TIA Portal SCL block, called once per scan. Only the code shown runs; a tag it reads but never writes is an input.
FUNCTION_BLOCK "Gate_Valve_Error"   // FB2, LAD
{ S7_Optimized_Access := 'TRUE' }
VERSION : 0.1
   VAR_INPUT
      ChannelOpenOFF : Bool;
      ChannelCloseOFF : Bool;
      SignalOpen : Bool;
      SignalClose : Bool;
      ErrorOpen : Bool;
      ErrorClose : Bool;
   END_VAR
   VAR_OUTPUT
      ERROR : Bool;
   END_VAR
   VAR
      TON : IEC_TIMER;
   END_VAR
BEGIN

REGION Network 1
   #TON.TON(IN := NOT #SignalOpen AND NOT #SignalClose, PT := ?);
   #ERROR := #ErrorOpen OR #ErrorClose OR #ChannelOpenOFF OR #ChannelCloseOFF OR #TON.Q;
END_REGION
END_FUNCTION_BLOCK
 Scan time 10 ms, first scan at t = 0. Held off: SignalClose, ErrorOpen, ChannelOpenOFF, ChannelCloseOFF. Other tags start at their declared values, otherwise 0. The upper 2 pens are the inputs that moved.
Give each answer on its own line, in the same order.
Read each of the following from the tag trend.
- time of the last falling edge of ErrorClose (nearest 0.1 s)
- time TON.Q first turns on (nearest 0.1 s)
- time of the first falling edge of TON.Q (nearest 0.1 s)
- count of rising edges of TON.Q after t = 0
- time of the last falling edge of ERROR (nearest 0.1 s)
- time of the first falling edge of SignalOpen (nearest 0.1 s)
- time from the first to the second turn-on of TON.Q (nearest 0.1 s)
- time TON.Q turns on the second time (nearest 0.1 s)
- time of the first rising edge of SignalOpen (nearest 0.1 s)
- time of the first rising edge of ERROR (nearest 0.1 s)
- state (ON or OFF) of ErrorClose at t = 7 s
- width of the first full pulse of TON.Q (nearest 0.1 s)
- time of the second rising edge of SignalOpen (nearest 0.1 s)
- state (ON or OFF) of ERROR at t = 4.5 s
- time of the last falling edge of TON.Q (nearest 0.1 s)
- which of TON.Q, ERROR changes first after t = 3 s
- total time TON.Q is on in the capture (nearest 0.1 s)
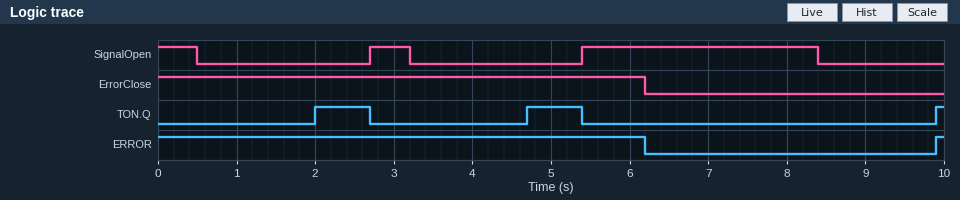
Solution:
6.2 s
2.0 s
2.7 s
3
6.2 s
0.5 s
2.7 s
4.7 s
2.7 s
9.9 s
OFF
0.7 s
5.4 s
ON
5.4 s
TON.Q
1.5 s
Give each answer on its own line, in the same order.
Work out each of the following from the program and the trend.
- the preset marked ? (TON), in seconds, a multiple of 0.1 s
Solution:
1.5 s
